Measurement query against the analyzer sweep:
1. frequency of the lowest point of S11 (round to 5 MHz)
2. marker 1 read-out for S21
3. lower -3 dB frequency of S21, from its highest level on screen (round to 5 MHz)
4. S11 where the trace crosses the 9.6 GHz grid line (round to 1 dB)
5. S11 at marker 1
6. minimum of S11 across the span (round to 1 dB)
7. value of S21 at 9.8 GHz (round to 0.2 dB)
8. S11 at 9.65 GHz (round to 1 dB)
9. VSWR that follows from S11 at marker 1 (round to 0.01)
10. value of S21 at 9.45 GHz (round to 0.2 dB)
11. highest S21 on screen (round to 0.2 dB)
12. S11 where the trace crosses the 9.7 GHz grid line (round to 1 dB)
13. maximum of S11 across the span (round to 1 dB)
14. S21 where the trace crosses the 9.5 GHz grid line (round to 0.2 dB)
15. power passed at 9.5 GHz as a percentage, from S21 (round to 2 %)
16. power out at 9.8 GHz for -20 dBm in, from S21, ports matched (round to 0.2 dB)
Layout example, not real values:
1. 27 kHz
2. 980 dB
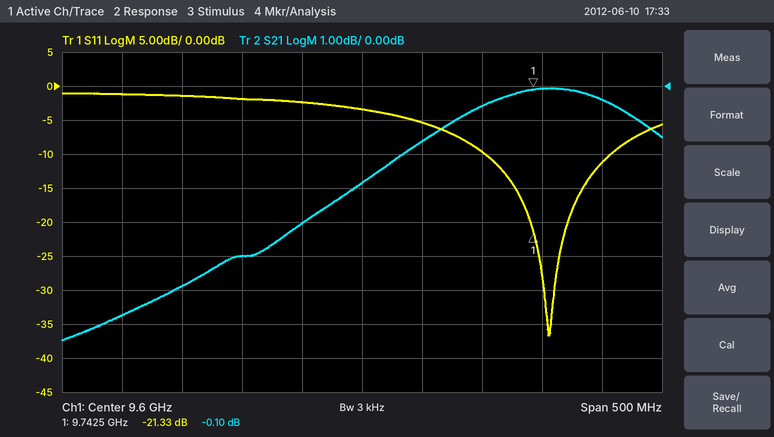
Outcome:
1. 9.755 GHz
2. -0.10 dB
3. 9.590 GHz
4. -3 dB
5. -21.33 dB
6. -37 dB
7. -0.4 dB
8. -5 dB
9. 1.19
10. -5.8 dB
11. 0.0 dB
12. -10 dB
13. -1 dB
14. -5.0 dB
15. 32 %
16. -20.4 dBm
